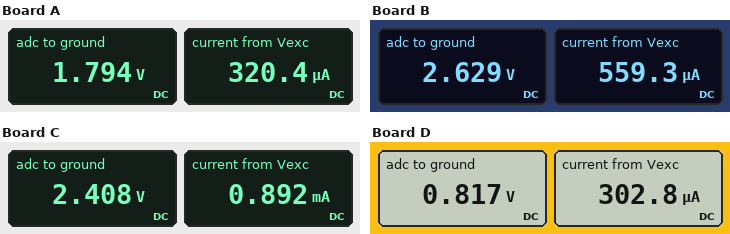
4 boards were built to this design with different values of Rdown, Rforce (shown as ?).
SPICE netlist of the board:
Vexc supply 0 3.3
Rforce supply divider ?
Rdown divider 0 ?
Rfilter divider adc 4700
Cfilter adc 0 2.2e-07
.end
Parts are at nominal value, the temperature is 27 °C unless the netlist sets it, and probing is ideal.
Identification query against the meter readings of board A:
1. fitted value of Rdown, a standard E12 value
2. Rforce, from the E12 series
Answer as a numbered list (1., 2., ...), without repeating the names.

1. 5.6 kΩ
2. 4.7 kΩ
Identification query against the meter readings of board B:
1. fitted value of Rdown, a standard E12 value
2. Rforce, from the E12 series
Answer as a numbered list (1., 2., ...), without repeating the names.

1. 4.7 kΩ
2. 1.2 kΩ
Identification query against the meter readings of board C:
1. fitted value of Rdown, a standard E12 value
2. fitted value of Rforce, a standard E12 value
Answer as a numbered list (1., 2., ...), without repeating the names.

1. 2.7 kΩ
2. 1 kΩ
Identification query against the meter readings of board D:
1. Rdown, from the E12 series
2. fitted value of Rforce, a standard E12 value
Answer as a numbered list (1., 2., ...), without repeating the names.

1. 2.7 kΩ
2. 8.2 kΩ
